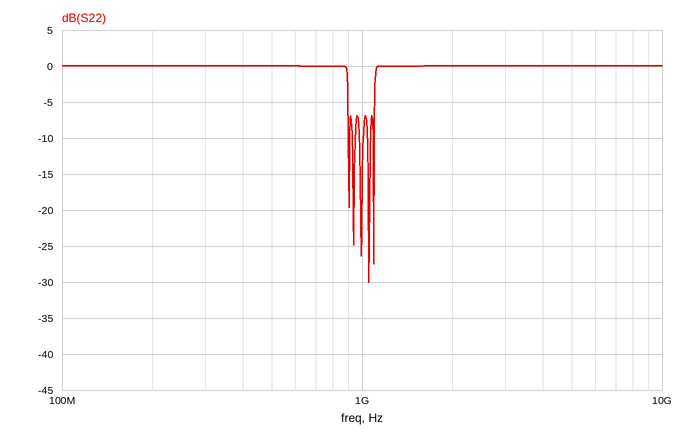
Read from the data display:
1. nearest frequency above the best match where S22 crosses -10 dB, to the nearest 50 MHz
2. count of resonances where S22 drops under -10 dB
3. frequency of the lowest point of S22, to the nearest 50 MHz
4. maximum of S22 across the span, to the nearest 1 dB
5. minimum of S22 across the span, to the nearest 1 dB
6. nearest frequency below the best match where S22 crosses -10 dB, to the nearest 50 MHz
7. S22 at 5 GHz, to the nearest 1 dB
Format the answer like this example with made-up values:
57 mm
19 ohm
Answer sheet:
1.05 GHz
5
1.05 GHz
0 dB
-30 dB
1.05 GHz
0 dB
